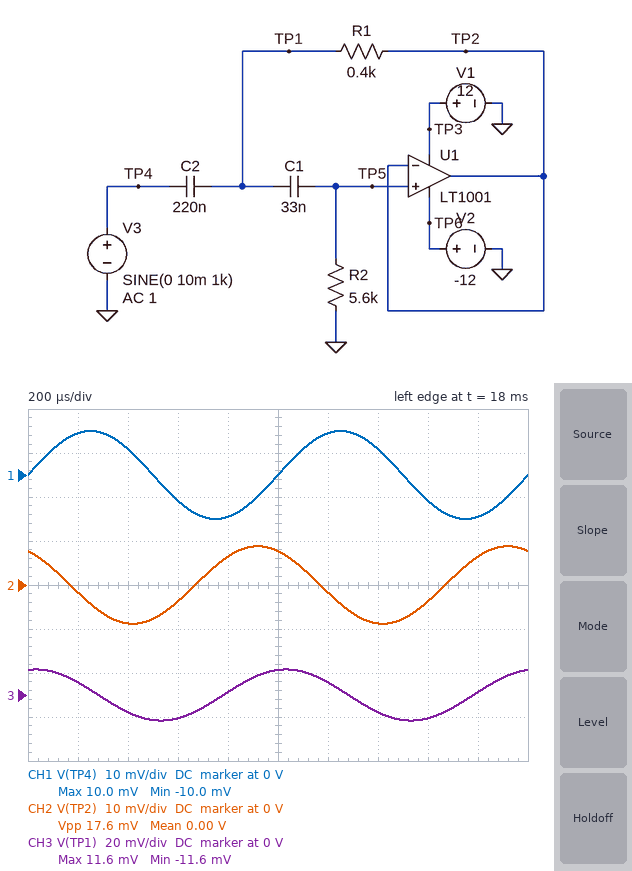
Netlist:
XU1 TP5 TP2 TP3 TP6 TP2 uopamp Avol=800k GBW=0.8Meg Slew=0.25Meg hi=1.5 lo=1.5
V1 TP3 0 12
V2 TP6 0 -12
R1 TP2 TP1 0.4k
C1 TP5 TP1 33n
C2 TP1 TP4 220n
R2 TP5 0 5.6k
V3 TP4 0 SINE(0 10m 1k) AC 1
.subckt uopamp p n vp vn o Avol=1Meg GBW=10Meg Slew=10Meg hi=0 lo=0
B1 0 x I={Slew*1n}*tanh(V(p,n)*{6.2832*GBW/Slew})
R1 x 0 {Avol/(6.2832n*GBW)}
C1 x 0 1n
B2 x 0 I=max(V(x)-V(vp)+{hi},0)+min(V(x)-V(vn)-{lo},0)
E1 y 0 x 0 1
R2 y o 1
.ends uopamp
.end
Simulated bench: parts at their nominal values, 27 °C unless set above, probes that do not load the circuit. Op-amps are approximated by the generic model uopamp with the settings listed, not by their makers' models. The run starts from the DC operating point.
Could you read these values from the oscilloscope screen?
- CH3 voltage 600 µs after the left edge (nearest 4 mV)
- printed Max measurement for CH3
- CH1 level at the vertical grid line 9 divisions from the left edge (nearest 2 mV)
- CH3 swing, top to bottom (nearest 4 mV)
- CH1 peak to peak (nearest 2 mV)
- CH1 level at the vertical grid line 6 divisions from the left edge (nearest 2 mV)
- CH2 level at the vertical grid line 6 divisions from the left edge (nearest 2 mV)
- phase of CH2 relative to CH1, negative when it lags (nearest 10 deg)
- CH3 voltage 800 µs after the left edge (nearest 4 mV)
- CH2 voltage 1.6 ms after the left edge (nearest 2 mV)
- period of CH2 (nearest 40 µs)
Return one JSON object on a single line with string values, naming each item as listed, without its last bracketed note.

{"CH3 voltage 600 µs after the left edge": "-12 mV", "printed Max measurement for CH3": "11.6 mV", "CH1 level at the vertical grid line 9 divisions from the left edge": "-10 mV", "CH3 swing, top to bottom": "24 mV", "CH1 peak to peak": "20 mV", "CH1 level at the vertical grid line 6 divisions from the left edge": "10 mV", "CH2 level at the vertical grid line 6 divisions from the left edge": "-2 mV", "phase of CH2 relative to CH1, negative when it lags": "120 deg", "CH3 voltage 800 µs after the left edge": "0 V", "CH2 voltage 1.6 ms after the left edge": "-4 mV", "period of CH2": "1.00 ms"}
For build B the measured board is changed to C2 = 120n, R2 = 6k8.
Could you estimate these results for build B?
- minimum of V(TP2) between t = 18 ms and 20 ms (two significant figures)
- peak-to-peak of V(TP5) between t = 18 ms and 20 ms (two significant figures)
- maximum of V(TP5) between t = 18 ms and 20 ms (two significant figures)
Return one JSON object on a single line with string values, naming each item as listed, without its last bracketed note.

{"minimum of V(TP2) between t = 18 ms and 20 ms": "-6.2 mV", "peak-to-peak of V(TP5) between t = 18 ms and 20 ms": "12 mV", "maximum of V(TP5) between t = 18 ms and 20 ms": "6.2 mV"}
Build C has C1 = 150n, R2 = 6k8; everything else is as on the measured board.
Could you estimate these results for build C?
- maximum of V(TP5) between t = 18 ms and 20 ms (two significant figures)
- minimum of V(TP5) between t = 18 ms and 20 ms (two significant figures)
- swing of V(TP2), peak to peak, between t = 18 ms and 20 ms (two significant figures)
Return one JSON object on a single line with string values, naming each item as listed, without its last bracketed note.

{"maximum of V(TP5) between t = 18 ms and 20 ms": "13 mV", "minimum of V(TP5) between t = 18 ms and 20 ms": "-13 mV", "swing of V(TP2), peak to peak, between t = 18 ms and 20 ms": "26 mV"}
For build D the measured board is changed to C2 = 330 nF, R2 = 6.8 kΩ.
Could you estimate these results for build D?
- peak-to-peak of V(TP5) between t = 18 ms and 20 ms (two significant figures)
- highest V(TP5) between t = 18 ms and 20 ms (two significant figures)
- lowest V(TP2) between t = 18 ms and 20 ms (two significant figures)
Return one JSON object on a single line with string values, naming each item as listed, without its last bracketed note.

{"peak-to-peak of V(TP5) between t = 18 ms and 20 ms": "25 mV", "highest V(TP5) between t = 18 ms and 20 ms": "13 mV", "lowest V(TP2) between t = 18 ms and 20 ms": "-13 mV"}
